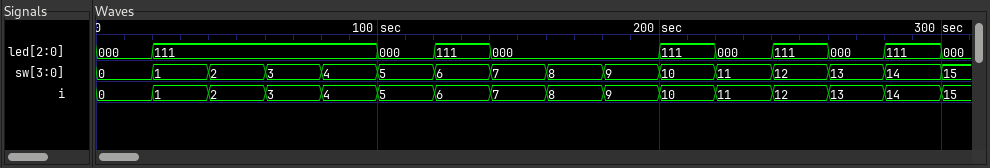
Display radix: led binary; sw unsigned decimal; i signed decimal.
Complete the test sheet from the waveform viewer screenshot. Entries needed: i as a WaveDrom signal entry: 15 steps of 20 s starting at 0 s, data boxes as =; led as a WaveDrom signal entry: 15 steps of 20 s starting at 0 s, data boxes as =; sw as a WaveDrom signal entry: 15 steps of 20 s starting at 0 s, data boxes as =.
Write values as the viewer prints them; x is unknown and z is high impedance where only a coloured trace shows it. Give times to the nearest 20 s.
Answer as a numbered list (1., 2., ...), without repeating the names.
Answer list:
1. {name: 'i', wave: '===============', data: '0 1 2 3 4 5 6 7 8 9 10 11 12 13 14'}
2. {name: 'led', wave: '==...===..=====', data: '000 111 000 111 000 111 000 111 000 111'}
3. {name: 'sw', wave: '===============', data: '0 1 2 3 4 5 6 7 8 9 10 11 12 13 14'}
